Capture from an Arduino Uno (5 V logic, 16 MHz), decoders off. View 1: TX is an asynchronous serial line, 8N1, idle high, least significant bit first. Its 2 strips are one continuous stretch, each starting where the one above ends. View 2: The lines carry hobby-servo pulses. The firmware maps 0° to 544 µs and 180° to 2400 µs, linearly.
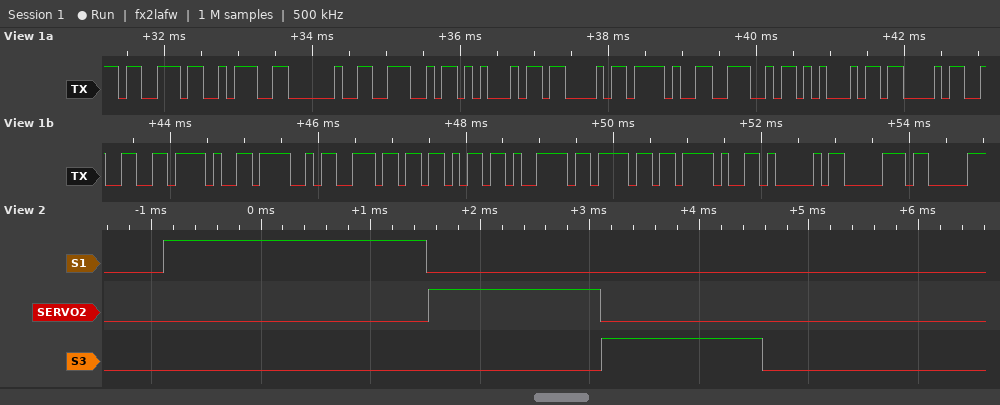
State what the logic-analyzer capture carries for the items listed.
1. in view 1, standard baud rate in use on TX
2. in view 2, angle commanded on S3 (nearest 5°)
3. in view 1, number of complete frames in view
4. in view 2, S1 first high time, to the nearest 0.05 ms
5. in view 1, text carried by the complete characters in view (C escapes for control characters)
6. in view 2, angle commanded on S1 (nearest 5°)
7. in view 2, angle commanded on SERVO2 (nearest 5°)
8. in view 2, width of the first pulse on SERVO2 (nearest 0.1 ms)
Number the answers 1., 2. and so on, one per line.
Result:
1. 9600 baud
2. 90°
3. 20
4. 2.40 ms
5. "s: NEC/NEC2/Onkyo/Ap"
6. 180°
7. 100°
8. 1.6 ms
